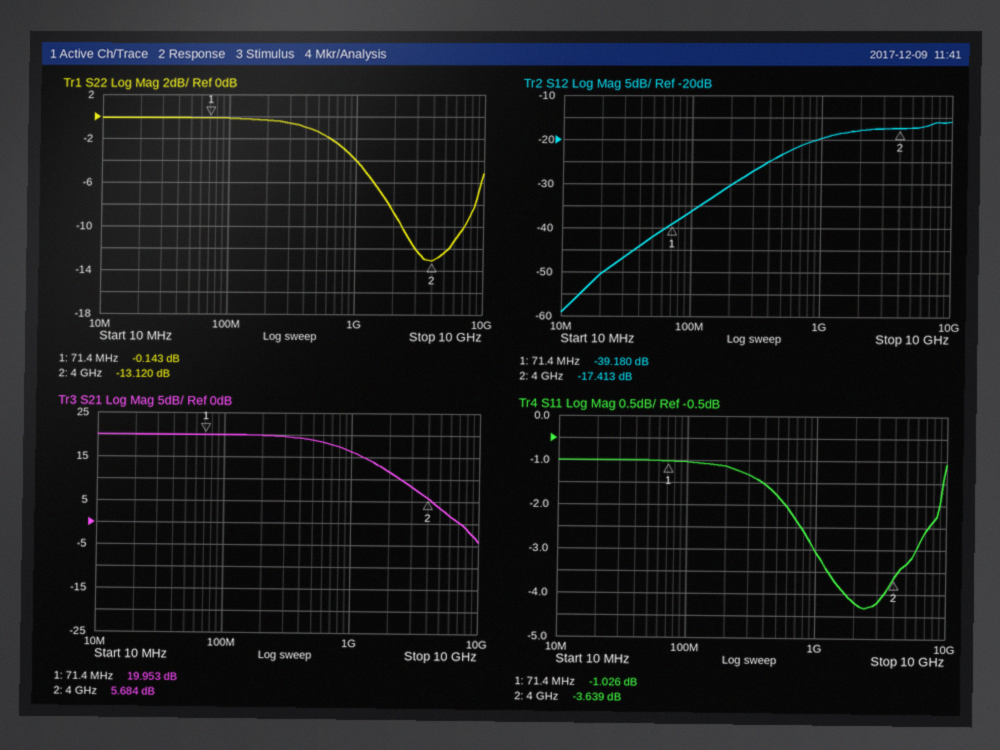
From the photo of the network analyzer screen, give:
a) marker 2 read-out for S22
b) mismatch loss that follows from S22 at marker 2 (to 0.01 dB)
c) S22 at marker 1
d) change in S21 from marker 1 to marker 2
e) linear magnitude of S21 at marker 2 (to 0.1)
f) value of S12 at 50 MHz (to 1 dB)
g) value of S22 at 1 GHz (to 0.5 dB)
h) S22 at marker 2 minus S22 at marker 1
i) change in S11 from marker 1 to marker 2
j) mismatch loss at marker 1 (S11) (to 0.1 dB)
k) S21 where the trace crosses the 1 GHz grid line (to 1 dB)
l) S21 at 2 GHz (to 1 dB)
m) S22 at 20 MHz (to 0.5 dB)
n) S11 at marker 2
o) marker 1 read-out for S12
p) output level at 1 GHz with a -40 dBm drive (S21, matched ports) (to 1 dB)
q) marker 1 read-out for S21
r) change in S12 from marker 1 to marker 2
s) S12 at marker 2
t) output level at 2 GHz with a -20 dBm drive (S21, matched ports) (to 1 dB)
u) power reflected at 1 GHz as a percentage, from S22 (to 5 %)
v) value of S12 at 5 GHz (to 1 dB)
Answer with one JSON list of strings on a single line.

["-13.120 dB", "0.22 dB", "-0.143 dB", "-14.269 dB", "1.9", "-42 dB", "-4.0 dB", "-12.977 dB", "-2.613 dB", "6.8 dB", "16 dB", "12 dB", "0.0 dB", "-3.639 dB", "-39.180 dB", "-24 dBm", "19.953 dB", "21.767 dB", "-17.413 dB", "-8 dBm", "40 %", "-17 dB"]
